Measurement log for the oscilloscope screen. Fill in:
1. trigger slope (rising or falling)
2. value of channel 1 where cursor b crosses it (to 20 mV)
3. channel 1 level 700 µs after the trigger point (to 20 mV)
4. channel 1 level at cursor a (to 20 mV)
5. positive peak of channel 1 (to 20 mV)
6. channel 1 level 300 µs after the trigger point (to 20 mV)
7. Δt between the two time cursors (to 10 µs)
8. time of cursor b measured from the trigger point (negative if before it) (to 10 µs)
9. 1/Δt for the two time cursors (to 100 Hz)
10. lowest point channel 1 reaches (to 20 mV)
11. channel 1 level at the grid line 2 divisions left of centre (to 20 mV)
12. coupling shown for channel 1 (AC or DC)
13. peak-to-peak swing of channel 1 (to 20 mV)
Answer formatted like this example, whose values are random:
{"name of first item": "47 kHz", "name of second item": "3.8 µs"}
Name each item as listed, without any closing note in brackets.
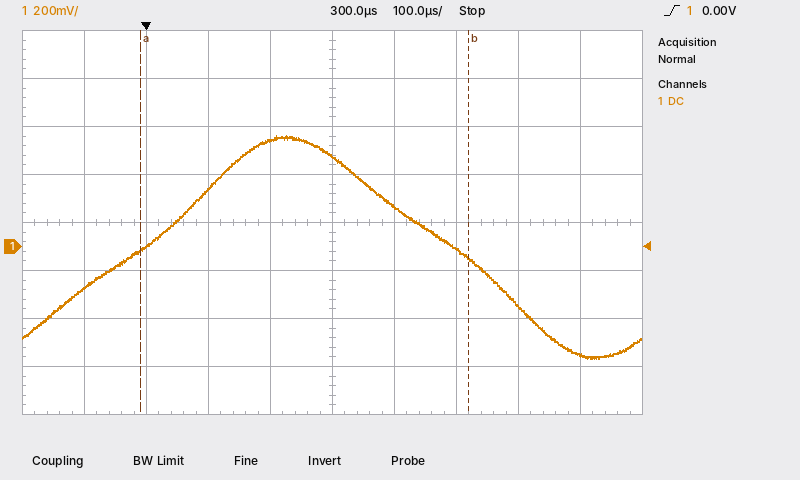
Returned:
{"trigger slope": "rising", "value of channel 1 where cursor b crosses it": "-40 mV", "channel 1 level 700 µs after the trigger point": "-460 mV", "channel 1 level at cursor a": "-20 mV", "positive peak of channel 1": "460 mV", "channel 1 level 300 µs after the trigger point": "380 mV", "Δt between the two time cursors": "530 µs", "time of cursor b measured from the trigger point (negative if before it)": "+520 µs", "1/Δt for the two time cursors": "1.9 kHz", "lowest point channel 1 reaches": "-460 mV", "channel 1 level at the grid line 2 divisions left of centre": "240 mV", "coupling shown for channel 1": "DC", "peak-to-peak swing of channel 1": "920 mV"}
